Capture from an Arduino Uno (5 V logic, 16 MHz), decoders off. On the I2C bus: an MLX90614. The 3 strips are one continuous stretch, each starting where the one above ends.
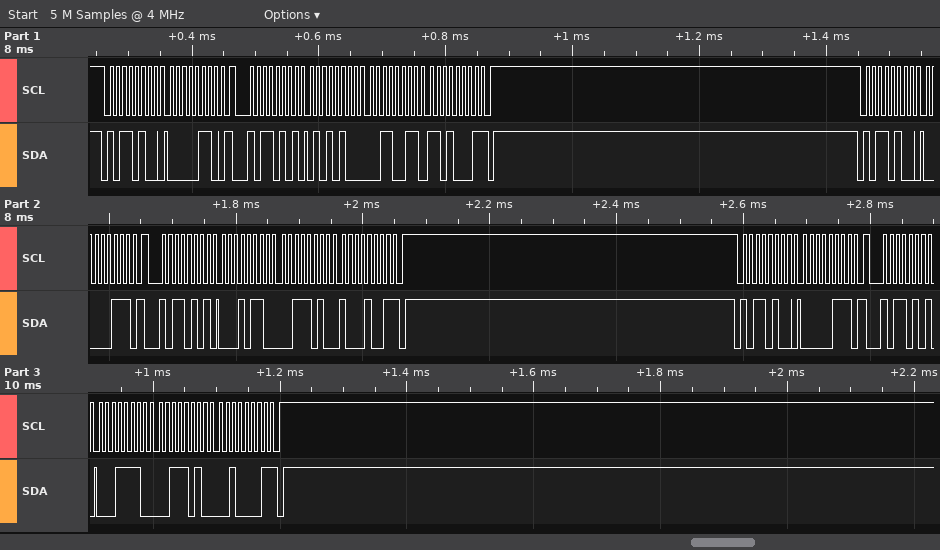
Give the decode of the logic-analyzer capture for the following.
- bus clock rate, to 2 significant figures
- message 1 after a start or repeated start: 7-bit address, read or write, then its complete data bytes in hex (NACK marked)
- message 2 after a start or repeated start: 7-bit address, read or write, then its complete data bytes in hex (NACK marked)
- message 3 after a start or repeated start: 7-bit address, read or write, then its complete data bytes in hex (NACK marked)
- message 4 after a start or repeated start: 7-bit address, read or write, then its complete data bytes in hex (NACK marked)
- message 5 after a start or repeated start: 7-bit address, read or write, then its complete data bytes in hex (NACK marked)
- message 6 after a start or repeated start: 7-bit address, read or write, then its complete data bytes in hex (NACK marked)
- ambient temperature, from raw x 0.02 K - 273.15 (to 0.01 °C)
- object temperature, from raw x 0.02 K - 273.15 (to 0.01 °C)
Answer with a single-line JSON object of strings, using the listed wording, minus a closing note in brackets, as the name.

{"bus clock rate, to 2 significant figures": "100 kHz", "message 1 after a start or repeated start: 7-bit address, read or write, then its complete data bytes in hex": "0x5A write: 06", "message 2 after a start or repeated start: 7-bit address, read or write, then its complete data bytes in hex": "0x5A read: 54 33 D1 NACK", "message 3 after a start or repeated start: 7-bit address, read or write, then its complete data bytes in hex": "0x5A write: 07", "message 4 after a start or repeated start: 7-bit address, read or write, then its complete data bytes in hex": "0x5A read: 16 3A 89 NACK", "message 5 after a start or repeated start: 7-bit address, read or write, then its complete data bytes in hex": "0x5A write: 07", "message 6 after a start or repeated start: 7-bit address, read or write, then its complete data bytes in hex": "0x5A read: 1E 3A 21 NACK", "ambient temperature, from raw x 0.02 K - 273.15": "-10.35 °C", "object temperature, from raw x 0.02 K - 273.15": "24.25 °C"}
